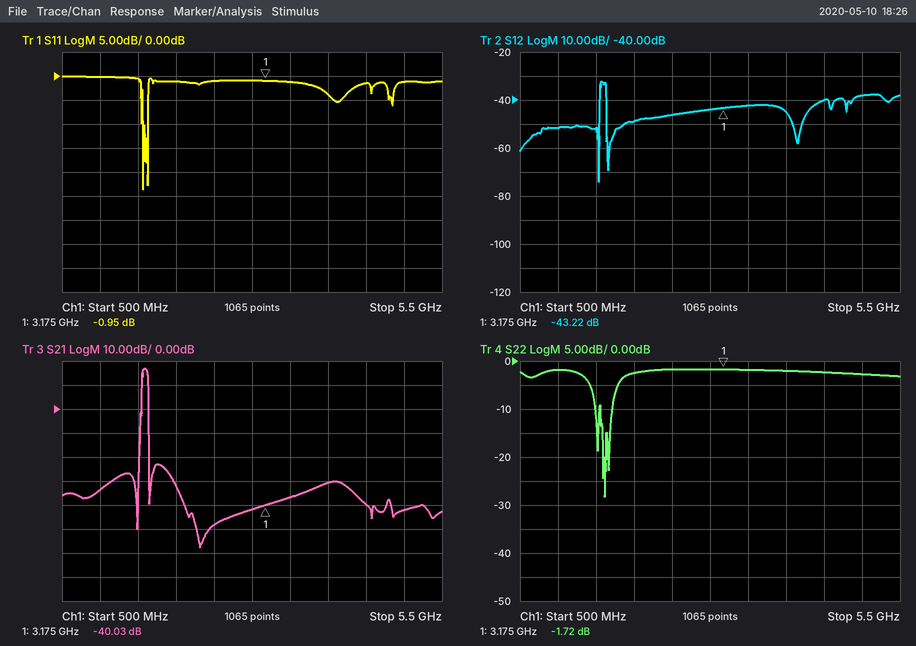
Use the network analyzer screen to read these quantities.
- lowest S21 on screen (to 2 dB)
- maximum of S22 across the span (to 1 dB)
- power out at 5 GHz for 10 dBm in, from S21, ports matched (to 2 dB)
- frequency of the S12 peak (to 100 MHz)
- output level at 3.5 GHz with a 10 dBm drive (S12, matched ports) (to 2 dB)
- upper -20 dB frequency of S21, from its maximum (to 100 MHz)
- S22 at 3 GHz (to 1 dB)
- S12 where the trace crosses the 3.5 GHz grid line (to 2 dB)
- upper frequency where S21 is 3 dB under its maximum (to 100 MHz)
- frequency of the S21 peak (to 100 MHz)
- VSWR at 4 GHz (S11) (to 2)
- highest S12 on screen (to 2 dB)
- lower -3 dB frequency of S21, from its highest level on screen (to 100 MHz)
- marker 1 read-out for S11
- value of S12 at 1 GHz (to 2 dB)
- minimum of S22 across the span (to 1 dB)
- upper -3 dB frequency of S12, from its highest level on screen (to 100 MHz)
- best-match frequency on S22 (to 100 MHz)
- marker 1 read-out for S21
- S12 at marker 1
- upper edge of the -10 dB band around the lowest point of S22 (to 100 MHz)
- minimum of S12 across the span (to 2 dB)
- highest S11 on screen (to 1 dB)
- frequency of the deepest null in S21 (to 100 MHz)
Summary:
-58 dB
-2 dB
-32 dBm
1.6 GHz
-32 dBm
1.6 GHz
-2 dB
-42 dB
1.6 GHz
1.6 GHz
4
-32 dB
1.6 GHz
-0.95 dB
-52 dB
-28 dB
1.6 GHz
1.6 GHz
-40.03 dB
-43.22 dB
1.7 GHz
-74 dB
0 dB
2.3 GHz
